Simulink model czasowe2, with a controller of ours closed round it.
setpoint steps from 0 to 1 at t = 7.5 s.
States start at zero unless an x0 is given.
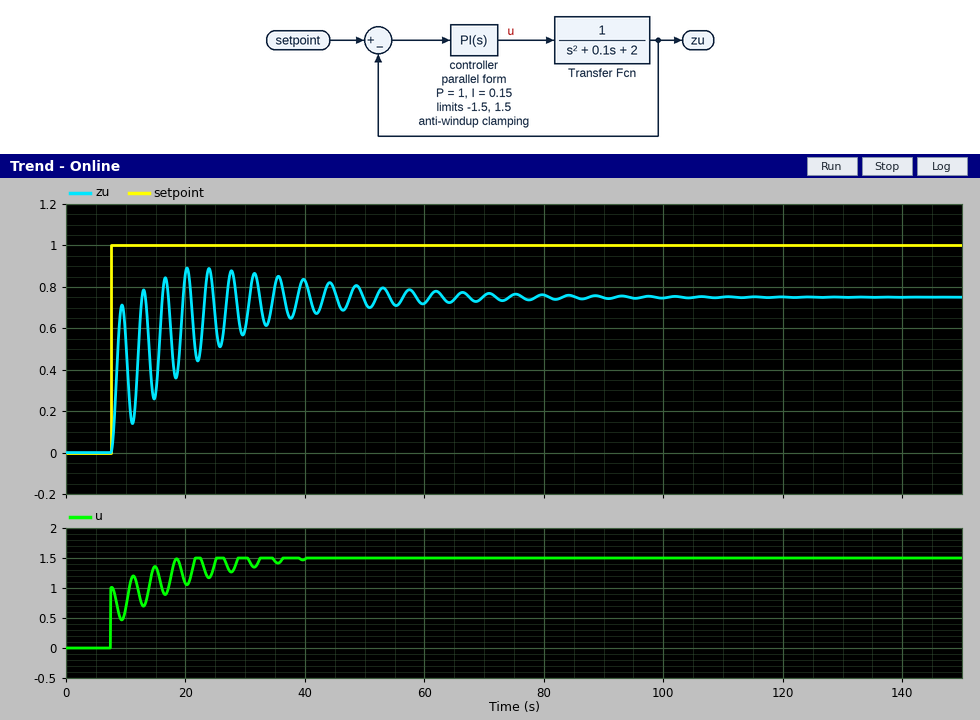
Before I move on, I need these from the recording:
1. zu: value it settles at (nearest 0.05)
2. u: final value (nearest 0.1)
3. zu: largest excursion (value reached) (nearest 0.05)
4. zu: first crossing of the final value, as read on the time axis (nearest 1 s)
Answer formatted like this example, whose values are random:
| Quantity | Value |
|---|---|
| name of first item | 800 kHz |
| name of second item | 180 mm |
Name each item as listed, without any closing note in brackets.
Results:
| Quantity | Value |
|---|---|
| zu: value it settles at | 0.75 |
| u: final value | 1.5 |
| zu: largest excursion (value reached) | 0.90 |
| zu: first crossing of the final value, as read on the time axis | 13 s |
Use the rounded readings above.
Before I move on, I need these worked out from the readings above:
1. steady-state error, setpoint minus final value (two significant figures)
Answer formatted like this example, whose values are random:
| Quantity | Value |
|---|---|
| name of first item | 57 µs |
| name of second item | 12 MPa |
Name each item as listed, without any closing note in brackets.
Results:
| Quantity | Value |
|---|---|
| steady-state error, setpoint minus final value | 0.25 |
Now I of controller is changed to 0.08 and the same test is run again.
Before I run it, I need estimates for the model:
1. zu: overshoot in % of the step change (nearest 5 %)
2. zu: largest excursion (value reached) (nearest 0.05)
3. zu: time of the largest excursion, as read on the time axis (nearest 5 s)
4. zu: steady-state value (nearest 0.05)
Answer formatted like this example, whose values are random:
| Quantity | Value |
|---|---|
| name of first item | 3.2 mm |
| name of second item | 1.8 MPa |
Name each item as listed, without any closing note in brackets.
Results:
| Quantity | Value |
|---|---|
| zu: overshoot in % of the step change | 10 % |
| zu: largest excursion (value reached) | 0.80 |
| zu: time of the largest excursion, as read on the time axis | 40 s |
| zu: steady-state value | 0.75 |
